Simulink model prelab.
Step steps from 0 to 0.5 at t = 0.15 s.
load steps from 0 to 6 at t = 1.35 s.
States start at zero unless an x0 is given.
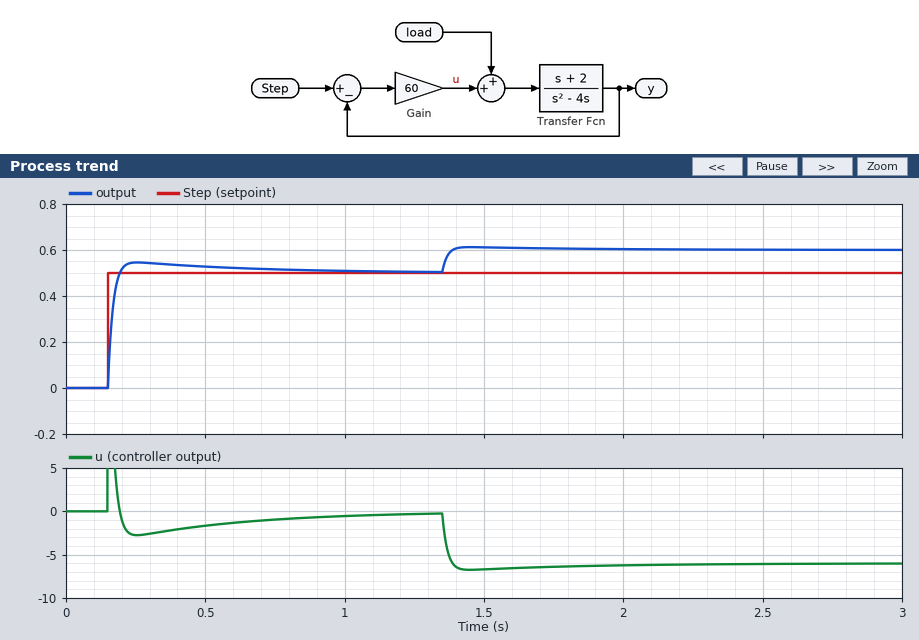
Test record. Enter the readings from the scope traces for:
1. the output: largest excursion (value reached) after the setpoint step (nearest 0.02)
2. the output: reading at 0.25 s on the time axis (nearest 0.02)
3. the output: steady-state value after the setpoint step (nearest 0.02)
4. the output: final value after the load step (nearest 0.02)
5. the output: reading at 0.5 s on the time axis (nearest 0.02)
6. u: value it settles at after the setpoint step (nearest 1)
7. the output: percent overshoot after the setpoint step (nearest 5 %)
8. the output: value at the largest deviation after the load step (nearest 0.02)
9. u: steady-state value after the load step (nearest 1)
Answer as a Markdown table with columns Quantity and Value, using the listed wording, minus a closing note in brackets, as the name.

| Quantity | Value |
|---|---|
| the output: largest excursion (value reached) after the setpoint step | 0.54 |
| the output: reading at 0.25 s on the time axis | 0.54 |
| the output: steady-state value after the setpoint step | 0.50 |
| the output: final value after the load step | 0.60 |
| the output: reading at 0.5 s on the time axis | 0.52 |
| u: value it settles at after the setpoint step | 0 |
| the output: percent overshoot after the setpoint step | 10 % |
| the output: value at the largest deviation after the load step | 0.62 |
| u: steady-state value after the load step | -6 |
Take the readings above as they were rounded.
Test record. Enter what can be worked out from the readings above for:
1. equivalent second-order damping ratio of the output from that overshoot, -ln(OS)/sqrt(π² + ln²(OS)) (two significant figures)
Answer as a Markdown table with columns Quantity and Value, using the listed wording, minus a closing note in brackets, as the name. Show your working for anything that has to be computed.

| Quantity | Value |
|---|---|
| equivalent second-order damping ratio of the output from that overshoot, -ln(OS)/sqrt(π² + ln²(OS)) | ln(0.1) = -2.303; 2.303 / sqrt(9.870 + 5.302) = 0.59 |
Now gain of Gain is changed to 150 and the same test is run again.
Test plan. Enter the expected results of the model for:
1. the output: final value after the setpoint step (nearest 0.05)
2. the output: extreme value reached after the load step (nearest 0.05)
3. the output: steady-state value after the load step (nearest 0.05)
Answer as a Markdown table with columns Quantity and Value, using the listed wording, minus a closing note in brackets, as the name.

| Quantity | Value |
|---|---|
| the output: final value after the setpoint step | 0.50 |
| the output: extreme value reached after the load step | 0.55 |
| the output: steady-state value after the load step | 0.55 |
